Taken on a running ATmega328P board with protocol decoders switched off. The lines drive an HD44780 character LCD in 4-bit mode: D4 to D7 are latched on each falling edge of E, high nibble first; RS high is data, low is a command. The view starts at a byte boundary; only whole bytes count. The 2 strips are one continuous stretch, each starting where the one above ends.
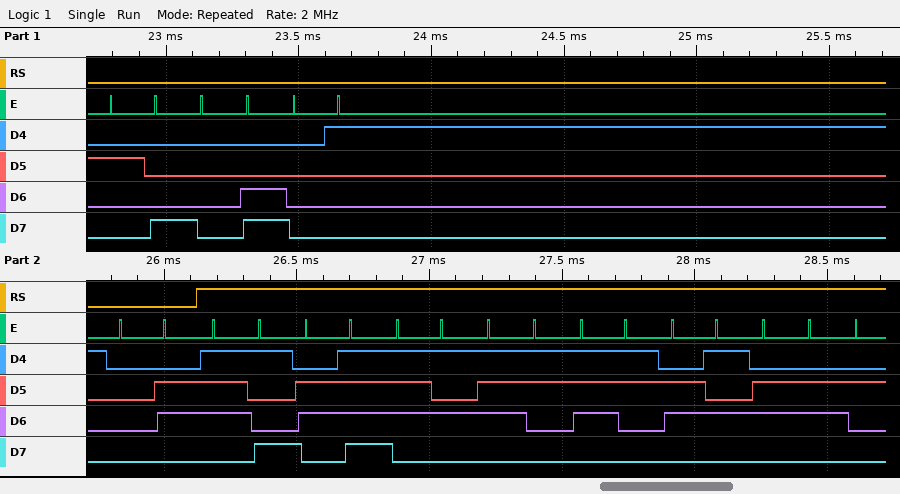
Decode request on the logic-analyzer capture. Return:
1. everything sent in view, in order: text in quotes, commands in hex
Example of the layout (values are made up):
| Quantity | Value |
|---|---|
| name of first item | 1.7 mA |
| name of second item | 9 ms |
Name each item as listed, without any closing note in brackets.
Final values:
| Quantity | Value |
|---|---|
| everything sent in view, in order: text in quotes, commands in hex | 0x28 0x0C 0x01 0x06 "youssef" |
